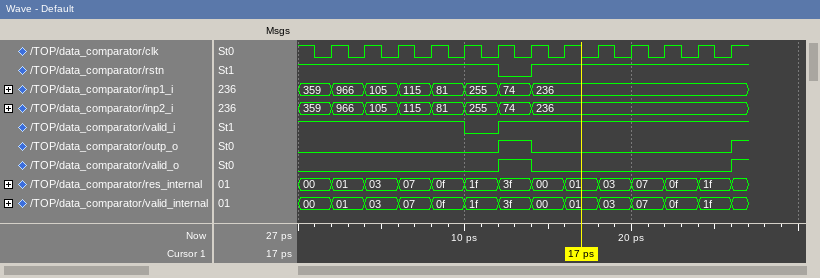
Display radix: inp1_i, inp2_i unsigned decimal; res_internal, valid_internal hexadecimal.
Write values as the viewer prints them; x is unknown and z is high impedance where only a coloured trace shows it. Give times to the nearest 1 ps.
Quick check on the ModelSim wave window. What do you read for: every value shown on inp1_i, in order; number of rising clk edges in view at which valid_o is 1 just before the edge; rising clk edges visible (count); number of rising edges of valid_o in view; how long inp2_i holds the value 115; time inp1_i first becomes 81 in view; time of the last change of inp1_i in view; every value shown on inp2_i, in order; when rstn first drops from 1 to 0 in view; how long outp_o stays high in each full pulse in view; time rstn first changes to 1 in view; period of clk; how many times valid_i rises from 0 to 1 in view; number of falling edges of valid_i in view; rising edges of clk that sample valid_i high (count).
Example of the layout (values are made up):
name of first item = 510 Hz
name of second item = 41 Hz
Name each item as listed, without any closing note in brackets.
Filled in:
every value shown on inp1_i, in order = 359, 966, 105, 115, 81, 255, 74, 236
number of rising clk edges in view at which valid_o is 1 just before the edge = 1
rising clk edges visible = 13
number of rising edges of valid_o in view = 2
how long inp2_i holds the value 115 = 2 ps
time inp1_i first becomes 81 in view = 8 ps
time of the last change of inp1_i in view = 14 ps
every value shown on inp2_i, in order = 359, 966, 105, 115, 81, 255, 74, 236
when rstn first drops from 1 to 0 in view = 12 ps
how long outp_o stays high in each full pulse in view = 2 ps
time rstn first changes to 1 in view = 14 ps
period of clk = 2 ps
how many times valid_i rises from 0 to 1 in view = 1
number of falling edges of valid_i in view = 1
rising edges of clk that sample valid_i high = 12
